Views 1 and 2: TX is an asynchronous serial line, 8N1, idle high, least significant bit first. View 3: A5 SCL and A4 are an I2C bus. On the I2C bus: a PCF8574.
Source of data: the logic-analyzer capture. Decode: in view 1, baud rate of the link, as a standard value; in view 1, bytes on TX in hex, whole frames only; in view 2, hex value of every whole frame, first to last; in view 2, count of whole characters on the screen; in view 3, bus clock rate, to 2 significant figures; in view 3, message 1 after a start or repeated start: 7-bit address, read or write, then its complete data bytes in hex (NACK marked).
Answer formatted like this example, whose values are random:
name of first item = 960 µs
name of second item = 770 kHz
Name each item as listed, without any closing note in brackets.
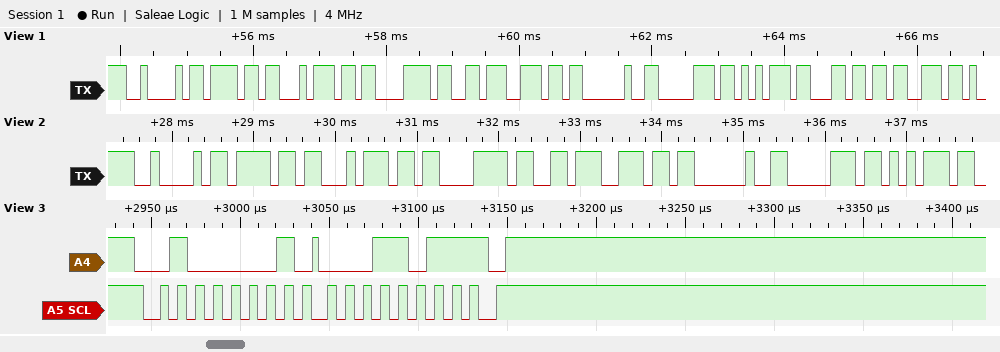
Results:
in view 1, baud rate of the link, as a standard value = 9600 baud
in view 1, bytes on TX in hex, whole frames only = 42 6F 74 C3 B3 6E 20 70 75 6C 73
in view 2, hex value of every whole frame, first to last = 42 6F 74 C3 B3 6E 20 70 75
in view 2, count of whole characters on the screen = 9
in view 3, bus clock rate, to 2 significant figures = 100 kHz
in view 3, message 1 after a start or repeated start: 7-bit address, read or write, then its complete data bytes in hex = 0x20 read: 1B NACK
